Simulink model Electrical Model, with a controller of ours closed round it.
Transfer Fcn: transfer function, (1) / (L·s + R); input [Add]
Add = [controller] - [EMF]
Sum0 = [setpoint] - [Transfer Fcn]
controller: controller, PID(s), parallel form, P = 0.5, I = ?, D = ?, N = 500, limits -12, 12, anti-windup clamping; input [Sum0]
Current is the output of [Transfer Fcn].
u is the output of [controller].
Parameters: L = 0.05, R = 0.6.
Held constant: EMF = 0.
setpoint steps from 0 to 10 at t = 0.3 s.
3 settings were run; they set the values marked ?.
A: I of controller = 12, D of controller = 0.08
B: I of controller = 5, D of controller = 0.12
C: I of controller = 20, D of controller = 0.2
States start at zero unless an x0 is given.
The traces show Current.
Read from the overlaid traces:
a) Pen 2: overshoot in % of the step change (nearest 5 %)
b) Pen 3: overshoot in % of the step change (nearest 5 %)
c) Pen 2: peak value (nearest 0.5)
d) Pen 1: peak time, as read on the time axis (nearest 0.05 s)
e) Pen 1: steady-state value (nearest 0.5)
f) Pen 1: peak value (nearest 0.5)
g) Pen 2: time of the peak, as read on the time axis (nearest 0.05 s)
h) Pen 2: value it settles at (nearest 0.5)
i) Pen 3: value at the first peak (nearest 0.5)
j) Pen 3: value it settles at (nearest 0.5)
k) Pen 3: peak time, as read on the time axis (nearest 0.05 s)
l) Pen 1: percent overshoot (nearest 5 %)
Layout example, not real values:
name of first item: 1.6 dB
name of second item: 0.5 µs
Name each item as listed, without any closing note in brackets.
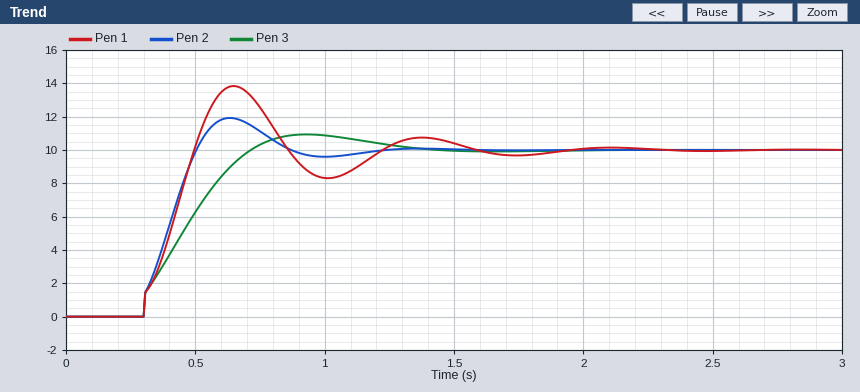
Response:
Pen 2: overshoot in % of the step change: 20 %
Pen 3: overshoot in % of the step change: 10 %
Pen 2: peak value: 12.0
Pen 1: peak time, as read on the time axis: 0.65 s
Pen 1: steady-state value: 10.0
Pen 1: peak value: 14.0
Pen 2: time of the peak, as read on the time axis: 0.65 s
Pen 2: value it settles at: 10.0
Pen 3: value at the first peak: 11.0
Pen 3: value it settles at: 10.0
Pen 3: peak time, as read on the time axis: 0.95 s
Pen 1: percent overshoot: 40 %
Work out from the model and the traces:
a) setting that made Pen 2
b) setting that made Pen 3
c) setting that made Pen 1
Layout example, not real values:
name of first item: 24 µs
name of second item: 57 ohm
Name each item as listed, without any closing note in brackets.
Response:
setting that made Pen 2: A
setting that made Pen 3: B
setting that made Pen 1: C
